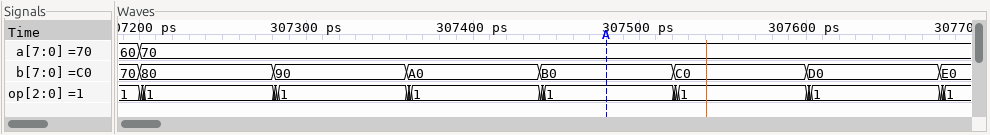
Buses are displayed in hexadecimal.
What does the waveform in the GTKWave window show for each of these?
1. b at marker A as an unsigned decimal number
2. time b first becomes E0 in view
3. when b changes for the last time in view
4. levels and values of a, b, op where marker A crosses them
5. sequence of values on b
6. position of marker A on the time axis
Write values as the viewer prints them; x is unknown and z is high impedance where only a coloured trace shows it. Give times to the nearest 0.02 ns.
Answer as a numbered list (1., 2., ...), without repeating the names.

1. 176
2. 307.68 ns
3. 307.68 ns
4. a=70, b=B0, op=1
5. 70, 80, 90, A0, B0, C0, D0, E0
6. 307.48 ns
